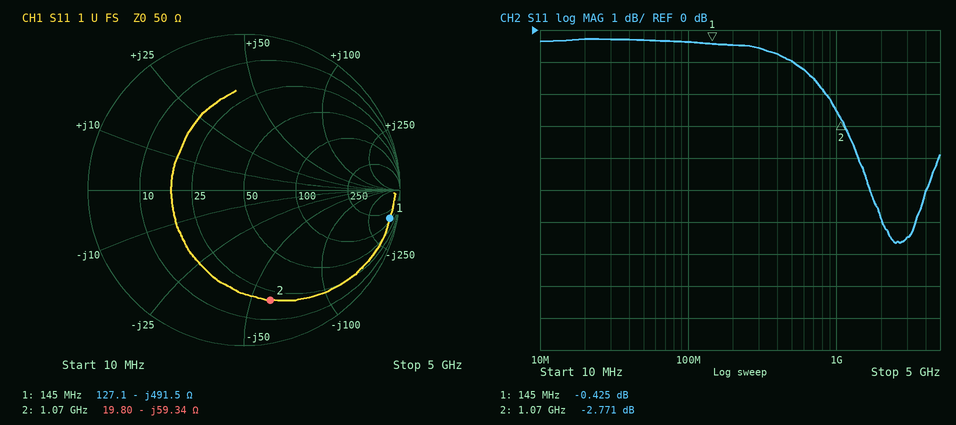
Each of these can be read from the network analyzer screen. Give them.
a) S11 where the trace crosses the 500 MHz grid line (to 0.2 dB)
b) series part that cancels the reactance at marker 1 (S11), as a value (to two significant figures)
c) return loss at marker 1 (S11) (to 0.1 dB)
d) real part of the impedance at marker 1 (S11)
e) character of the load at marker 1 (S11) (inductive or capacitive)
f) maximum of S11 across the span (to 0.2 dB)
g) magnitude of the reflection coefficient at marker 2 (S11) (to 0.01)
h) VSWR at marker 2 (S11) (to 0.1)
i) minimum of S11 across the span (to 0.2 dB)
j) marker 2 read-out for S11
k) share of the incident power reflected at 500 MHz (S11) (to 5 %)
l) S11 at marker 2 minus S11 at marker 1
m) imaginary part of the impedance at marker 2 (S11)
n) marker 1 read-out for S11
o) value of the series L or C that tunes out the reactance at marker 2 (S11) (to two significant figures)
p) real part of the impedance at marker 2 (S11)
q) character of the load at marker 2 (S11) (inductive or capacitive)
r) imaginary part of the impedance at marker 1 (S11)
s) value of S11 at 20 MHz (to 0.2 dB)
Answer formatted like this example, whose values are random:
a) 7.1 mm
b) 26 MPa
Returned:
a) -1.0 dB
b) 540 nH
c) 0.4 dB
d) 127.1 Ω
e) capacitive
f) -0.2 dB
g) 0.73
h) 6.3
i) -6.6 dB
j) -2.771 dB
k) 80 %
l) -2.346 dB
m) -59.34 Ω
n) -0.425 dB
o) 8.8 nH
p) 19.80 Ω
q) capacitive
r) -491.5 Ω
s) -0.2 dB
